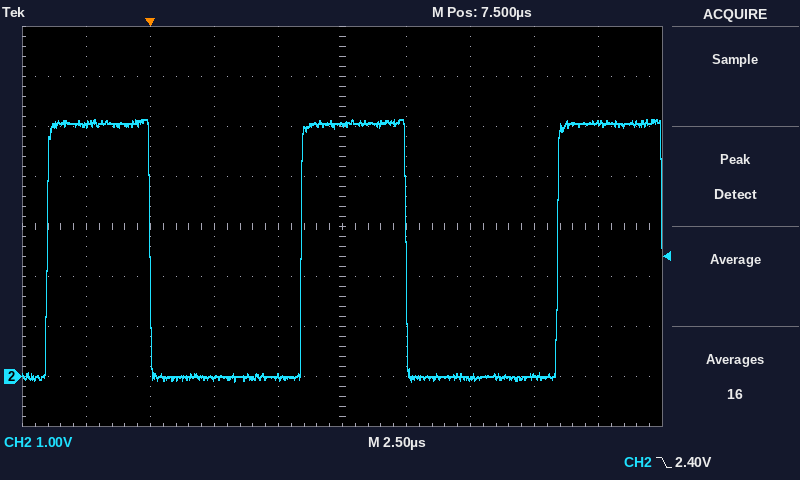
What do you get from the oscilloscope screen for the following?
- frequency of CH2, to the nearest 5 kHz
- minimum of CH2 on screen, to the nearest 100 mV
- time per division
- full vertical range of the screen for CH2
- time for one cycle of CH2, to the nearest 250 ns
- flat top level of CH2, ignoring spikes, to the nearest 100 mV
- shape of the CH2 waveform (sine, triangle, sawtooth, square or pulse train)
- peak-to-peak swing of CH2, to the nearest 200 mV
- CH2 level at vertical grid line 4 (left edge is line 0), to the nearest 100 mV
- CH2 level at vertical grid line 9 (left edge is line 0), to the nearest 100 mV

100 kHz
-100 mV
2.5 µs
8 V
10.00 µs
5.1 V
pulse train
5.2 V
0.0 V
5.1 V
